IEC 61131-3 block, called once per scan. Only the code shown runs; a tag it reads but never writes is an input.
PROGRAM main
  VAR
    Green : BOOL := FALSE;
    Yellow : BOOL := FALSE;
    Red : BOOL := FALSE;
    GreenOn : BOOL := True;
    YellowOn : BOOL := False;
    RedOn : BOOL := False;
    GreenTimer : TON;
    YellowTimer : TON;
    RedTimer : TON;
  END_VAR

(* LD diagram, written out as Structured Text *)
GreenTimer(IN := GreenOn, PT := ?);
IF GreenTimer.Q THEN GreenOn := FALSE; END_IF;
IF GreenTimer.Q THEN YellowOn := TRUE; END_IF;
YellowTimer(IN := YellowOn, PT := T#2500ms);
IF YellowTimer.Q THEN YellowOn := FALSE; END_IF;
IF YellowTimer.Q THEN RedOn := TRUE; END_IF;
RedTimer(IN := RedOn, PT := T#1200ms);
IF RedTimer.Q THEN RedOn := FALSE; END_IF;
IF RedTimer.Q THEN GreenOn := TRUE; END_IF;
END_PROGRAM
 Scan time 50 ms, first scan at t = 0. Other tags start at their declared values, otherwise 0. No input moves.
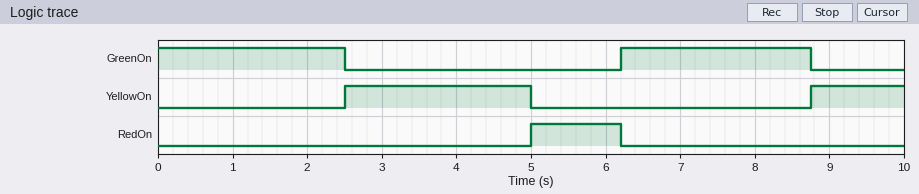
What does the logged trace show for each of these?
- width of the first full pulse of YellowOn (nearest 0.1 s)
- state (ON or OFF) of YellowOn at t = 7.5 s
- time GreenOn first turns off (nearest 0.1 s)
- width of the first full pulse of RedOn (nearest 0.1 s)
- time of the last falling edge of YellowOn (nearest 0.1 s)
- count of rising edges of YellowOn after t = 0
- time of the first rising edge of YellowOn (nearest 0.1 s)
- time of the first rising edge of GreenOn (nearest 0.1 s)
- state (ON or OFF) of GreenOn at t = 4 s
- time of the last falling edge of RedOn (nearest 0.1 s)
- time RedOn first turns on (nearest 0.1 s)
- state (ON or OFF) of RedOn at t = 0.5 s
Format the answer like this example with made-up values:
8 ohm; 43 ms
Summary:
2.5 s; OFF; 2.5 s; 1.2 s; 5.0 s; 2; 2.5 s; 6.2 s; OFF; 6.2 s; 5.0 s; OFF
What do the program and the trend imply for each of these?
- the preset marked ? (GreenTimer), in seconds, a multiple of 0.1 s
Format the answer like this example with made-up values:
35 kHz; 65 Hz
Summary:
2.5 s
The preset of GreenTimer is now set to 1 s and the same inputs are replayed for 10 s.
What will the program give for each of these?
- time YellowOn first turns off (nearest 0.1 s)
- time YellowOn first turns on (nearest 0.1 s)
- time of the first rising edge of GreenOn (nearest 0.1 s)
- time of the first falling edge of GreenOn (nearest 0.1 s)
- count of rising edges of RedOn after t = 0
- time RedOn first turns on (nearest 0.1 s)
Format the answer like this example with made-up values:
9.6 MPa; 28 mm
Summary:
3.5 s; 1.0 s; 4.7 s; 1.0 s; 2; 3.5 s
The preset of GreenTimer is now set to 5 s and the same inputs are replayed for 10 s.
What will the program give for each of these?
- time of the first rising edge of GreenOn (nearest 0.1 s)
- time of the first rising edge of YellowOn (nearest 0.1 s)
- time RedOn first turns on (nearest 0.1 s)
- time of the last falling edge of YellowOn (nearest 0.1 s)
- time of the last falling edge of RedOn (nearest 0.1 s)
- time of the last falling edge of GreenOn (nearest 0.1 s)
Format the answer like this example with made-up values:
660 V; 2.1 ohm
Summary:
8.7 s; 5.0 s; 7.5 s; 7.5 s; 8.7 s; 5.0 s
